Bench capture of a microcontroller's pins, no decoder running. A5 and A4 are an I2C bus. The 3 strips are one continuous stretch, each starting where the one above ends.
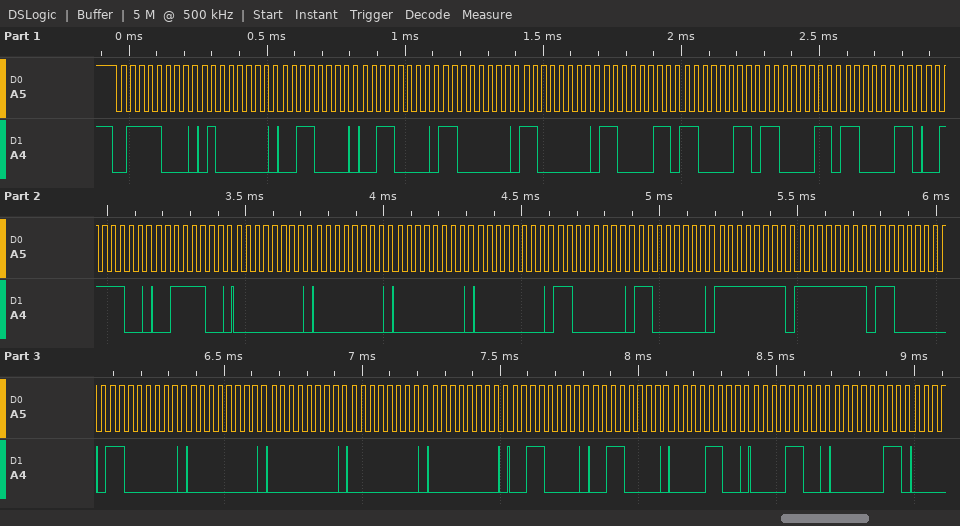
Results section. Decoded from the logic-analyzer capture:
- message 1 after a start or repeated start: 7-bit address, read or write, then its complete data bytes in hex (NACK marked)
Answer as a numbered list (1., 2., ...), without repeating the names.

1. 0x3C write: 40 30 30 C0 C0 C3 C3 C3 C3 3C 3C 00 00 00 00 C0 C0 FF FF C0 C0 00 00 00 00 30 30 0C 0C 03
